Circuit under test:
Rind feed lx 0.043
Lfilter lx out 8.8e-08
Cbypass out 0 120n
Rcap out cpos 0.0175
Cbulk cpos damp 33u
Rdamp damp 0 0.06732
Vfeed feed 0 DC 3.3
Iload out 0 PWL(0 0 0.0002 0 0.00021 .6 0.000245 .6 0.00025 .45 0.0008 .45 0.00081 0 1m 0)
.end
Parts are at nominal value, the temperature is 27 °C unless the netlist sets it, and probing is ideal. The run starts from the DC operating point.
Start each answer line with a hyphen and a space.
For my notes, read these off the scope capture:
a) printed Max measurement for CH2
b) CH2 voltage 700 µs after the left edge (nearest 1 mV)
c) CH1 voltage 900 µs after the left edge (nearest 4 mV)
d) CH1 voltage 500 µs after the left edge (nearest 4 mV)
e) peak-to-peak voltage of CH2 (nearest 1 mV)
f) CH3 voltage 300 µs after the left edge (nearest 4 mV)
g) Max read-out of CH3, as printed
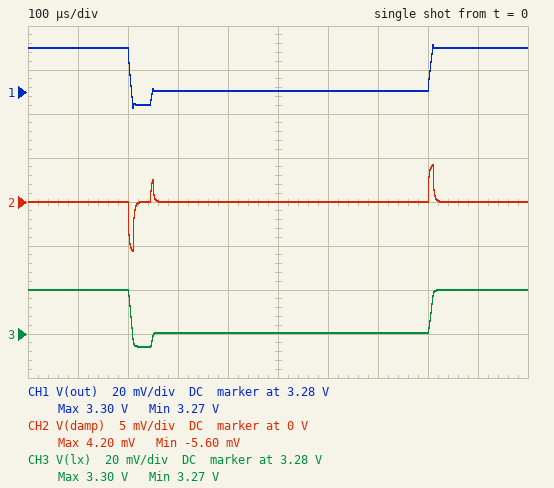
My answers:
- 4.20 mV
- 0 V
- 3.300 V
- 3.280 V
- 10 mV
- 3.280 V
- 3.30 V
